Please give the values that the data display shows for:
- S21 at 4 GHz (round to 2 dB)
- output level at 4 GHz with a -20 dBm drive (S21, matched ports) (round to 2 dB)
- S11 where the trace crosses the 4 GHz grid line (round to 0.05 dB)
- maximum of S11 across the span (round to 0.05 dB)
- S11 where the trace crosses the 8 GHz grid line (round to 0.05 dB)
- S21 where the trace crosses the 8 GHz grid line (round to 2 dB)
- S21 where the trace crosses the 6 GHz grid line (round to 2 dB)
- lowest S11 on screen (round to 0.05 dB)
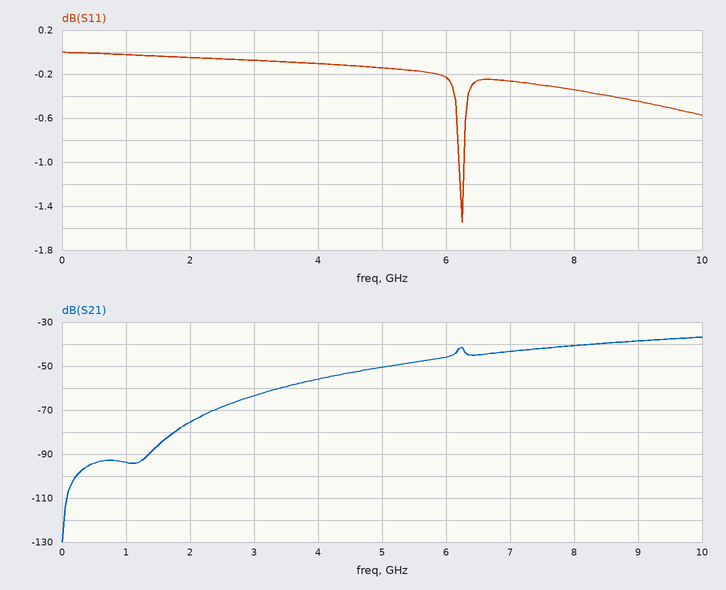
-56 dB
-76 dBm
-0.10 dB
0.00 dB
-0.35 dB
-40 dB
-46 dB
-1.55 dB
